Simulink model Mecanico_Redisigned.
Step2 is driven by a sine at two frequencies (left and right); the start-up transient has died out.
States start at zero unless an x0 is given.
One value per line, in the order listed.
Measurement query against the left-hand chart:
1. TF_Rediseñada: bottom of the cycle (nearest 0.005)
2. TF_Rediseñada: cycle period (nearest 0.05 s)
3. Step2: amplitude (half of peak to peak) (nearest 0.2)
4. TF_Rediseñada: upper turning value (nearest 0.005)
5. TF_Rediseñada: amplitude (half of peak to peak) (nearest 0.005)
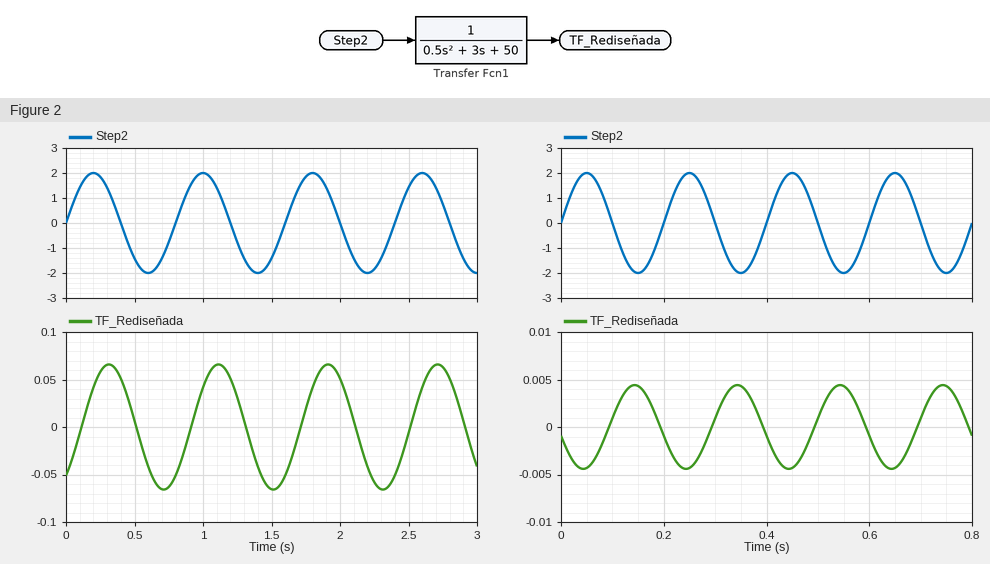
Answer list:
-0.065
0.80 s
2.0
0.065
0.065
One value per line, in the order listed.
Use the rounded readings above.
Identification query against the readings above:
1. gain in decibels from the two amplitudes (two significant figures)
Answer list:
-30 dB
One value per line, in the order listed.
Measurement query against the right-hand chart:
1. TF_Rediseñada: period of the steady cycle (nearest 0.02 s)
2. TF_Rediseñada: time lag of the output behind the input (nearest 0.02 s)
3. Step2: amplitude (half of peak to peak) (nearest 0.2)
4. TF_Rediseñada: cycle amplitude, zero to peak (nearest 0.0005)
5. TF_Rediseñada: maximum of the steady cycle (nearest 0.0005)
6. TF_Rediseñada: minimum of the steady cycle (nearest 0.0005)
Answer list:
0.20 s
0.10 s
2.0
0.0045
0.0045
-0.0045
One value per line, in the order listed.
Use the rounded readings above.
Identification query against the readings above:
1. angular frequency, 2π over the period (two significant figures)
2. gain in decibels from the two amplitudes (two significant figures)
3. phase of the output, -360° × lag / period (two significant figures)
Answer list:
31 rad/s
-53 dB
-180°
